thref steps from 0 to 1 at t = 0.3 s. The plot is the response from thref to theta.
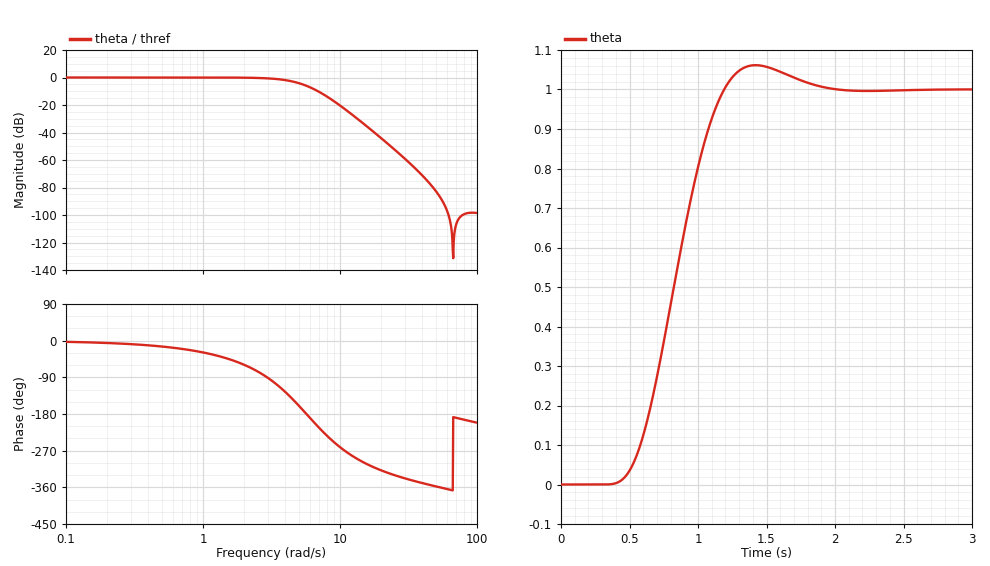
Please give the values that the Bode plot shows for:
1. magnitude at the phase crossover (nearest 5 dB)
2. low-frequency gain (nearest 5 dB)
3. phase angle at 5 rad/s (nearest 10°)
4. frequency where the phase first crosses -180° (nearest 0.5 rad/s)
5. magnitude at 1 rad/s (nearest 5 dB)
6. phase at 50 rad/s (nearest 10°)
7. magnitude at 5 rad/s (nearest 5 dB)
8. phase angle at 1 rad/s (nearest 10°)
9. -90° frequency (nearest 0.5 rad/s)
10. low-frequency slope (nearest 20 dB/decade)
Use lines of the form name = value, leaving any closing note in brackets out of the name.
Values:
magnitude at the phase crossover = -5 dB
low-frequency gain = 0 dB
phase angle at 5 rad/s = -160°
frequency where the phase first crosses -180° = 5.5 rad/s
magnitude at 1 rad/s = 0 dB
phase at 50 rad/s = -360°
magnitude at 5 rad/s = -5 dB
phase angle at 1 rad/s = -30°
-90° frequency = 3.0 rad/s
low-frequency slope = 0 dB/decade
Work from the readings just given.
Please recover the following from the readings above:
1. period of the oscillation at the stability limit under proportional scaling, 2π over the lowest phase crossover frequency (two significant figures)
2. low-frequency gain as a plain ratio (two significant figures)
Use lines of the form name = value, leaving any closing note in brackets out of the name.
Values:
period of the oscillation at the stability limit under proportional scaling, 2π over the lowest phase crossover frequency = 1.1 s
low-frequency gain as a plain ratio = 1.0
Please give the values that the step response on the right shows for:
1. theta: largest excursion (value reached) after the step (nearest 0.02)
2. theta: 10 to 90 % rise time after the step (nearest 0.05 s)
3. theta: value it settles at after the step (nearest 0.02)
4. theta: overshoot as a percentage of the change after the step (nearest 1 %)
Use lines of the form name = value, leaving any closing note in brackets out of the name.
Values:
theta: largest excursion (value reached) after the step = 1.06
theta: 10 to 90 % rise time after the step = 0.50 s
theta: value it settles at after the step = 1.00
theta: overshoot as a percentage of the change after the step = 6 %
